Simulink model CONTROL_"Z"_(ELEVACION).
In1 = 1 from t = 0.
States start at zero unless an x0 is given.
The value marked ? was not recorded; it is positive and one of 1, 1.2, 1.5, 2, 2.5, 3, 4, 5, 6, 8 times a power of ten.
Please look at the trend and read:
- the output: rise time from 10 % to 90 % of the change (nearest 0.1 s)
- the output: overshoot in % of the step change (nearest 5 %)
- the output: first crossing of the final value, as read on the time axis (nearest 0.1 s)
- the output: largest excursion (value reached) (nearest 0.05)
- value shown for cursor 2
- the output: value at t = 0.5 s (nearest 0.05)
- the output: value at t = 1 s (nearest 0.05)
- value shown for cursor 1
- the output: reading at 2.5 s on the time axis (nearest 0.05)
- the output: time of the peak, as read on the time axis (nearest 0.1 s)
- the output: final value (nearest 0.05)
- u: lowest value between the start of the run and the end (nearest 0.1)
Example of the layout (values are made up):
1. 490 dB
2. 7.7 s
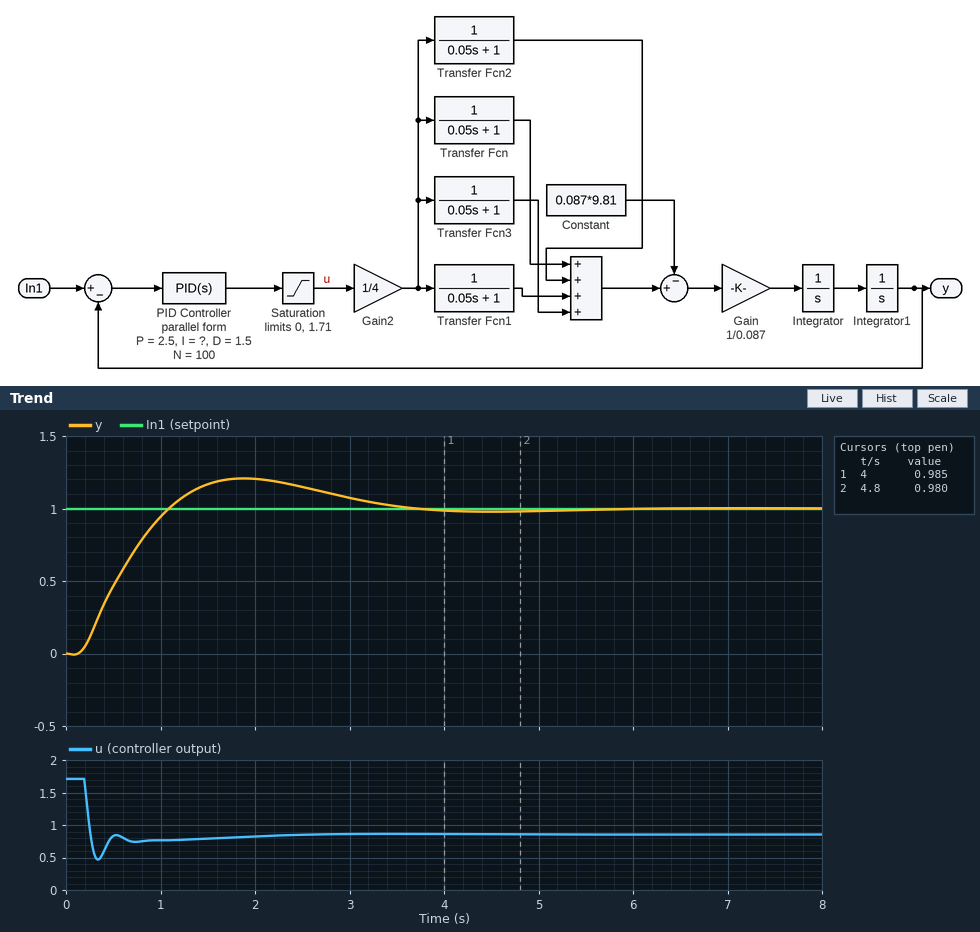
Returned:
1. 0.7 s
2. 20 %
3. 1.1 s
4. 1.20
5. 0.980
6. 0.45
7. 0.95
8. 0.985
9. 1.15
10. 1.9 s
11. 1.00
12. 0.5
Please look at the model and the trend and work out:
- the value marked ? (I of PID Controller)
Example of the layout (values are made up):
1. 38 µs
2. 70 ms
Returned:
1. 3
